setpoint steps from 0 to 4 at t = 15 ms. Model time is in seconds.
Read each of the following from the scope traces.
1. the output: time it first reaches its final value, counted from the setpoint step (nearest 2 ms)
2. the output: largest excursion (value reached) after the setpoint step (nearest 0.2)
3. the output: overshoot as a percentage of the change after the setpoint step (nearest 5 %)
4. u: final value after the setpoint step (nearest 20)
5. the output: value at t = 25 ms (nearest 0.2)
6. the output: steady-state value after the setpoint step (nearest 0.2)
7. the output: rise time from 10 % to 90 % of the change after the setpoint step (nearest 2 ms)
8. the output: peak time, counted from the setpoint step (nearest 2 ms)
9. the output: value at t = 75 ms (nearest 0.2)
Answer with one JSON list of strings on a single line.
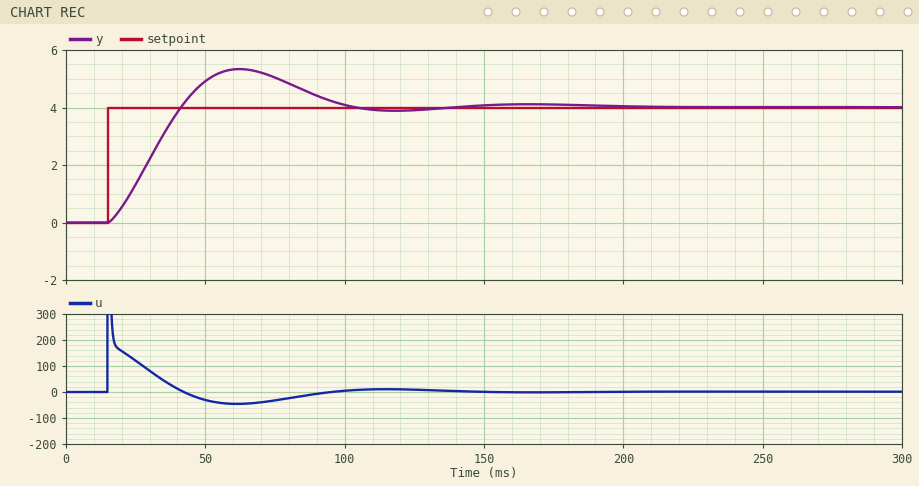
["26 ms", "5.4", "35 %", "0", "1.4", "4.0", "20 ms", "48 ms", "5.0"]
